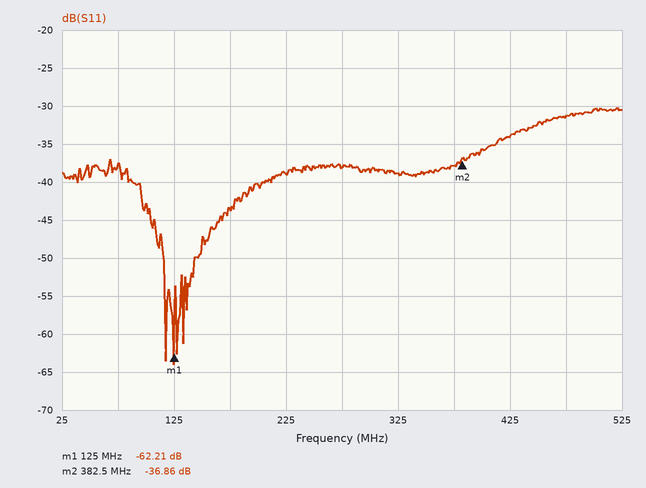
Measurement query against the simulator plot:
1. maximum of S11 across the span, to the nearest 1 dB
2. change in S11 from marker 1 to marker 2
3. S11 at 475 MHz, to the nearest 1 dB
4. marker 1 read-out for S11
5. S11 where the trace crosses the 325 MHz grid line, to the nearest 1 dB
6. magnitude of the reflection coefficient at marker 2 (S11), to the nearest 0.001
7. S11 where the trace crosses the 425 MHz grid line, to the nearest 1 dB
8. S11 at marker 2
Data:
-30 dB
25.35 dB
-31 dB
-62.21 dB
-39 dB
0.014
-34 dB
-36.86 dB
